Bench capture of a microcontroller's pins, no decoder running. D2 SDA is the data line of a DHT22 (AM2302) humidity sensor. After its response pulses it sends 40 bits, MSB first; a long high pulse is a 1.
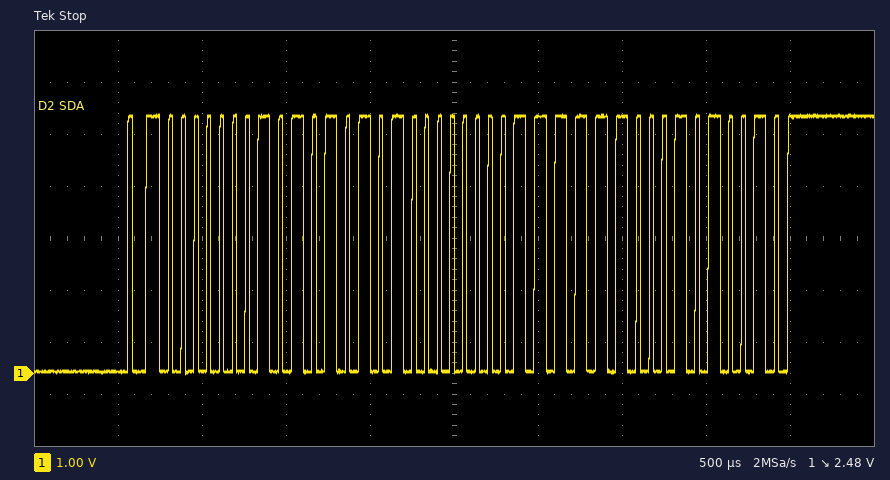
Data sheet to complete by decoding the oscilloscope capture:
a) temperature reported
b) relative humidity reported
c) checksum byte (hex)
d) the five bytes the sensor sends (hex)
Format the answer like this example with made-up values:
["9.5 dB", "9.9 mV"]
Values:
["25.2 °C", "34.1 %", "0x52", "01 55 00 FC 52"]
